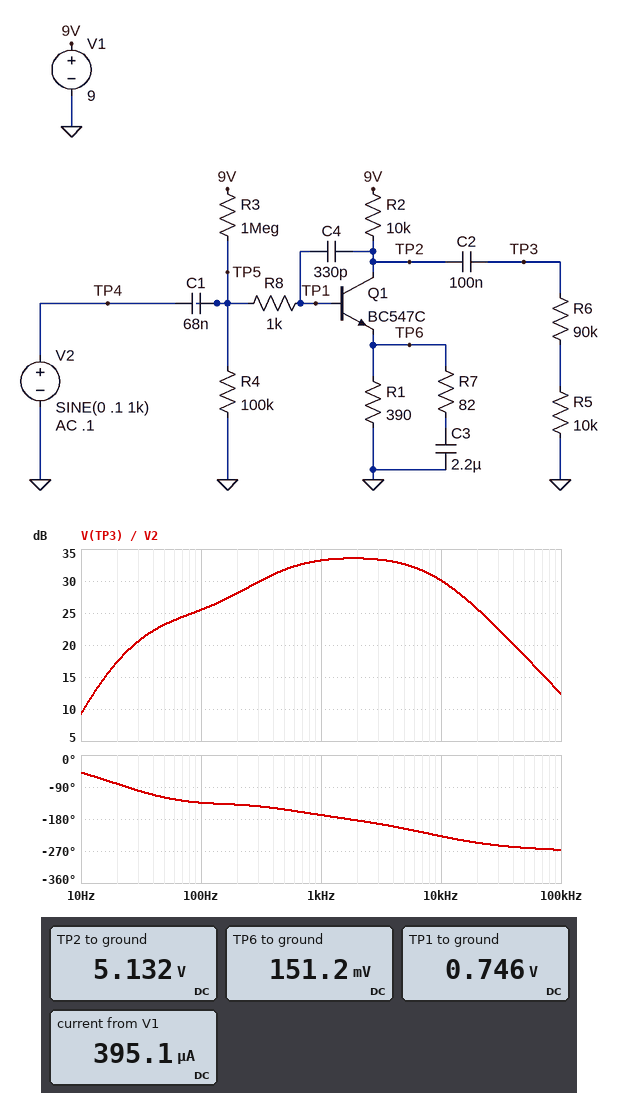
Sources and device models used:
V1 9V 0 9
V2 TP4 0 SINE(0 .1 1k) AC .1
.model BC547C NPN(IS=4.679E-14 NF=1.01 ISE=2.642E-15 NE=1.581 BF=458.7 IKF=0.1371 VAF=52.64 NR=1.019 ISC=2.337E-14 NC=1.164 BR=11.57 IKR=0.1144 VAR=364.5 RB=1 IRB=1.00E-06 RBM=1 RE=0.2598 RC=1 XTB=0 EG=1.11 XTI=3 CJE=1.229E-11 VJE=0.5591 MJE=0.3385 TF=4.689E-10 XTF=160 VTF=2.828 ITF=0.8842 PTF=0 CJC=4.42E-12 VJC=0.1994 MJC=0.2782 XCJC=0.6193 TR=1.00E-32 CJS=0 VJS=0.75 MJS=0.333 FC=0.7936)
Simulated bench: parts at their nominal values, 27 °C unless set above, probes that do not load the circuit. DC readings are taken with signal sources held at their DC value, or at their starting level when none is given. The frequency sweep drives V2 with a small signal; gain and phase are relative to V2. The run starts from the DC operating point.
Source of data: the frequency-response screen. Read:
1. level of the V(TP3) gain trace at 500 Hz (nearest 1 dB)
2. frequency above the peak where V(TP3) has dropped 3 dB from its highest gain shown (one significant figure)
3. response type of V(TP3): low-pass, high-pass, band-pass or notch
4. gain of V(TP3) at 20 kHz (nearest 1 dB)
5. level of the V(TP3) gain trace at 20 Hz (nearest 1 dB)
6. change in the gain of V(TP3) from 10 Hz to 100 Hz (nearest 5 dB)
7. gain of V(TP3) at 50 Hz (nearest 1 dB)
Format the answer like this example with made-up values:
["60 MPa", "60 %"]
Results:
["32 dB", "9 kHz", "band-pass", "26 dB", "17 dB", "15 dB", "23 dB"]
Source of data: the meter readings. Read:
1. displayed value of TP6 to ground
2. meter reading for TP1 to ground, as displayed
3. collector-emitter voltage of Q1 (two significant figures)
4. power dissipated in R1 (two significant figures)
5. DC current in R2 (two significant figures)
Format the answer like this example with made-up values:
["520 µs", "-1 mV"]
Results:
["151.2 mV", "0.746 V", "5.0 V", "59 µW", "390 µA"]
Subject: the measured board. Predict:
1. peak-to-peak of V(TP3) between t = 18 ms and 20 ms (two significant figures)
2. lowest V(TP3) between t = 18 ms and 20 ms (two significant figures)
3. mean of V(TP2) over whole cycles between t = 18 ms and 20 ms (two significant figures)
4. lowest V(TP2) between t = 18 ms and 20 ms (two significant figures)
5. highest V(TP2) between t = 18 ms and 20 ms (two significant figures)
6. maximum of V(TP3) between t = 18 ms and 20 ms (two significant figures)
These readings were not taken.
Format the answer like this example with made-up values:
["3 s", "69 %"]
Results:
["7.9 V", "-4.6 V", "5.0 V", "410 mV", "8.3 V", "3.3 V"]
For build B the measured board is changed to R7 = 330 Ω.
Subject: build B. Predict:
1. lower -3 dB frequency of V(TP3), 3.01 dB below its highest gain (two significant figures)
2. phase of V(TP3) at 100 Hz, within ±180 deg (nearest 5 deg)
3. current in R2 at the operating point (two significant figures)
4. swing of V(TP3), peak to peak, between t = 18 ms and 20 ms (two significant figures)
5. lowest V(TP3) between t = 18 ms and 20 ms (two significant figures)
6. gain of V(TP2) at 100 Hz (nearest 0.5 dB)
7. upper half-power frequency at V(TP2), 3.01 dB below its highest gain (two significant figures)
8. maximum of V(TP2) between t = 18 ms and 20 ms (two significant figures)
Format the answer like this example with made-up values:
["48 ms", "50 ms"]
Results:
["120 Hz", "-140 deg", "390 µA", "5.7 V", "-3.0 V", "26.0 dB", "13 kHz", "7.8 V"]
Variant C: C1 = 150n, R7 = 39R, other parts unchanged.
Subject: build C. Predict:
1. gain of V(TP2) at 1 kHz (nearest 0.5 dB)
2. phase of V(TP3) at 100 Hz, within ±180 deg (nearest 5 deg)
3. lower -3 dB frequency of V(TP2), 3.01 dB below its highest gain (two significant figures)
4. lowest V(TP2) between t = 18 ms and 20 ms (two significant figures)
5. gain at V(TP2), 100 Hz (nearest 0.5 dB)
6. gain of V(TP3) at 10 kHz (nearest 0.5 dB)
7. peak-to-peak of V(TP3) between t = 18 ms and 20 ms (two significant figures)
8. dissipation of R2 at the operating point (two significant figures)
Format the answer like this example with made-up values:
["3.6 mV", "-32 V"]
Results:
["36.0 dB", "-140 deg", "530 Hz", "230 mV", "26.5 dB", "31.5 dB", "8.4 V", "1.5 mW"]
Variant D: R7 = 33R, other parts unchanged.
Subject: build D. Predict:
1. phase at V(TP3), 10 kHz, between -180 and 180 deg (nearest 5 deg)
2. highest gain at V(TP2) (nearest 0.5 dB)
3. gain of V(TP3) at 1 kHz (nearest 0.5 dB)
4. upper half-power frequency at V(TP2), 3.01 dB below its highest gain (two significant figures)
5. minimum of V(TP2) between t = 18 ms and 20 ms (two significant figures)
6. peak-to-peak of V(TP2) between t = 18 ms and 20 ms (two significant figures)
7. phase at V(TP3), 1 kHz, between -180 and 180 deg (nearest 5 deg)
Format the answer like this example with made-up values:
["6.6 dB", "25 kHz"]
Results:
["125 deg", "35.5 dB", "34.5 dB", "7.8 kHz", "250 mV", "8.3 V", "-165 deg"]
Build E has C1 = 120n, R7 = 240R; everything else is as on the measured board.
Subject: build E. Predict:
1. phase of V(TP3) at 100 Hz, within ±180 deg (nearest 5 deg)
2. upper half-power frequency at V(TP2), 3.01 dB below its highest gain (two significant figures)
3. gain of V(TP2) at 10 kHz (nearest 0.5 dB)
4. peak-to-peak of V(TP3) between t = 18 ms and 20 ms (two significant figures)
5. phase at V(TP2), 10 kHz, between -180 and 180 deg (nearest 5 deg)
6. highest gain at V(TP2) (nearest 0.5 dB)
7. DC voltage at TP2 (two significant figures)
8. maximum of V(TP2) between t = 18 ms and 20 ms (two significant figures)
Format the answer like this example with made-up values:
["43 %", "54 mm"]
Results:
["-145 deg", "11 kHz", "28.5 dB", "6.6 V", "135 deg", "31.0 dB", "5.1 V", "8.0 V"]
